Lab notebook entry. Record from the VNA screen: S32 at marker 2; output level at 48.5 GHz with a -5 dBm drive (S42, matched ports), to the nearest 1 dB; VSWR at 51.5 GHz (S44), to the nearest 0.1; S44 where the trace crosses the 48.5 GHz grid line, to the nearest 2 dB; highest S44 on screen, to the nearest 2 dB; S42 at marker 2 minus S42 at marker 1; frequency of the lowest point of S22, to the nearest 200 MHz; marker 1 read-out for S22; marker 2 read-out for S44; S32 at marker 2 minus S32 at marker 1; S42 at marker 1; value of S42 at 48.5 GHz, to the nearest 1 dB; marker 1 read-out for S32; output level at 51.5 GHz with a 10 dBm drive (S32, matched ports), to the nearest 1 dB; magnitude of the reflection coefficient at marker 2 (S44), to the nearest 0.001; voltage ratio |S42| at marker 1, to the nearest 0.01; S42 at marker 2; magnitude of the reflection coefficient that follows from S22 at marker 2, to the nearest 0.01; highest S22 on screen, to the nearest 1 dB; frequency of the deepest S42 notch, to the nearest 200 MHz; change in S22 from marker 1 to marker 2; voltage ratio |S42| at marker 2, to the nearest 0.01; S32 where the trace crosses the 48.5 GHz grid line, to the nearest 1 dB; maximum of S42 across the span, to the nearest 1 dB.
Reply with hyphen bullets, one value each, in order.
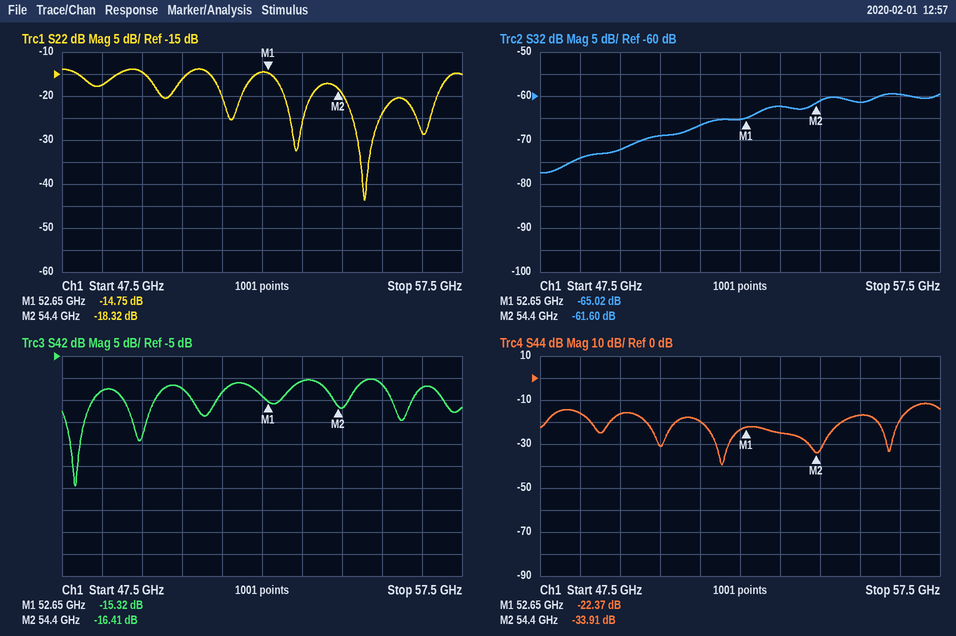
- -61.60 dB
- -18 dBm
- 1.2
- -16 dB
- -12 dB
- -1.09 dB
- 55.0 GHz
- -14.75 dB
- -33.91 dB
- 3.42 dB
- -15.32 dB
- -13 dB
- -65.02 dB
- -57 dBm
- 0.020
- 0.17
- -16.41 dB
- 0.12
- -14 dB
- 47.8 GHz
- -3.57 dB
- 0.15
- -74 dB
- -10 dB
